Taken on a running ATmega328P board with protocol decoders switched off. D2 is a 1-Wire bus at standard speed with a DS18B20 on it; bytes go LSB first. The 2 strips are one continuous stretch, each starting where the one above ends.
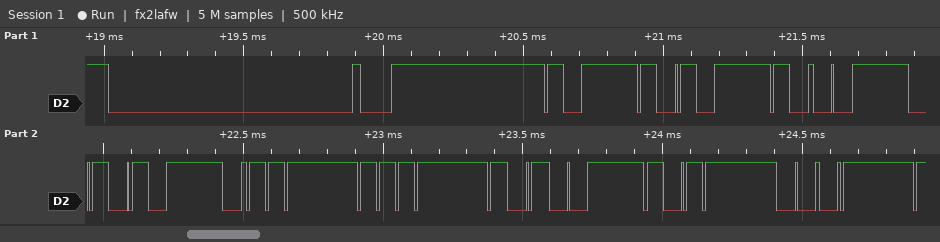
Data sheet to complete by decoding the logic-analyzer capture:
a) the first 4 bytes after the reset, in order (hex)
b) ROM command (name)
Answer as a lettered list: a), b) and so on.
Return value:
a) 55 28 FF D2
b) Match ROM
